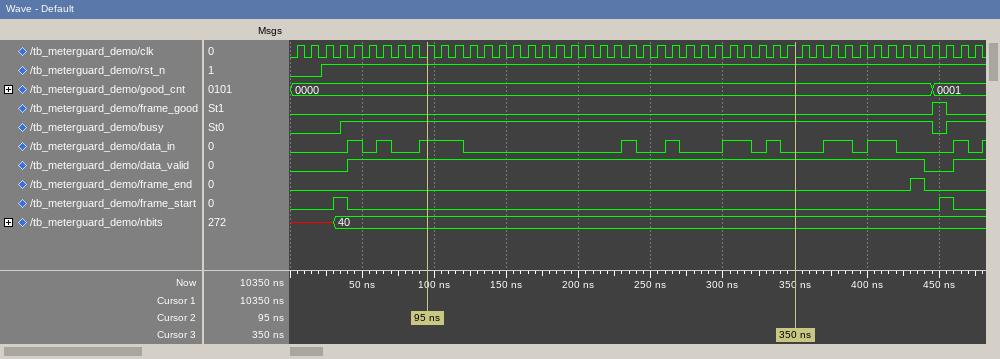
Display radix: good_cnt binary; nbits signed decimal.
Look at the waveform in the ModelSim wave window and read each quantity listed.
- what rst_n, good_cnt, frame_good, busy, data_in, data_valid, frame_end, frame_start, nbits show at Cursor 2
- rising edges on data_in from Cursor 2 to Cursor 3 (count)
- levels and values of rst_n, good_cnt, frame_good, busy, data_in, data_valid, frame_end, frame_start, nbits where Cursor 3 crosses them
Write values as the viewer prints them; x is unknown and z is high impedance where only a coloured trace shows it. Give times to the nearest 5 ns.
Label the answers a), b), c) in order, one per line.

a) rst_n=1, good_cnt=0000, frame_good=0, busy=1, data_in=1, data_valid=1, frame_end=0, frame_start=0, nbits=40
b) 4
c) rst_n=1, good_cnt=0000, frame_good=0, busy=1, data_in=0, data_valid=1, frame_end=0, frame_start=0, nbits=40
